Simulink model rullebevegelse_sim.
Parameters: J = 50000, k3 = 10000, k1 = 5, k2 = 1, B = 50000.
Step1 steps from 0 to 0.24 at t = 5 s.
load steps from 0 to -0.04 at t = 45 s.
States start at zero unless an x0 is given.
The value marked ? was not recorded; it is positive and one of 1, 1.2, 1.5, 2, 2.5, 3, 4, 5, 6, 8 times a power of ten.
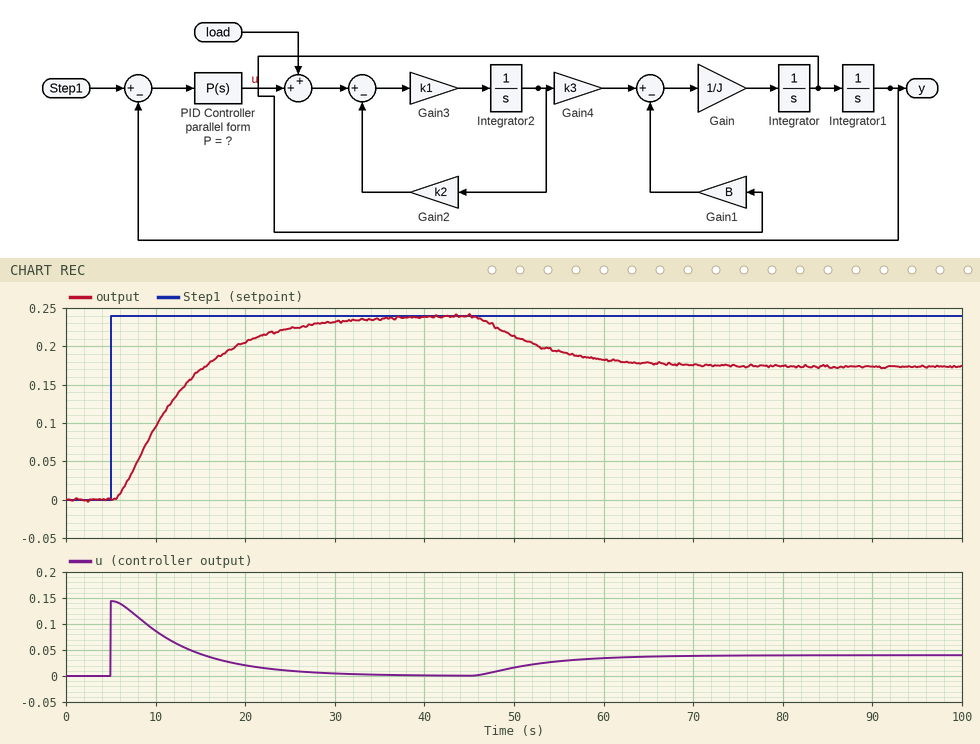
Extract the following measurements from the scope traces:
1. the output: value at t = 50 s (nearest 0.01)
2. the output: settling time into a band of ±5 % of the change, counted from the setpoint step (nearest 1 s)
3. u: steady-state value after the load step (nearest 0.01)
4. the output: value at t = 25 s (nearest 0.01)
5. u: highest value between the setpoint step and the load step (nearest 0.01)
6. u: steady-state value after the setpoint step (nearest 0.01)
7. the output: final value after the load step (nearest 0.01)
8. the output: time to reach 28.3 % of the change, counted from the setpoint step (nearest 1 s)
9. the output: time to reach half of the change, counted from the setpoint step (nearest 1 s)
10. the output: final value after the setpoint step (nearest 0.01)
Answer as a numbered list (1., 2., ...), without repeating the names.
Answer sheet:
1. 0.21
2. 22 s
3. 0.04
4. 0.22
5. 0.14
6. 0.00
7. 0.17
8. 4 s
9. 6 s
10. 0.24
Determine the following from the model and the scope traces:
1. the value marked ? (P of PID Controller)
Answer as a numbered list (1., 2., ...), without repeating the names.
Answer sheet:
1. 0.6
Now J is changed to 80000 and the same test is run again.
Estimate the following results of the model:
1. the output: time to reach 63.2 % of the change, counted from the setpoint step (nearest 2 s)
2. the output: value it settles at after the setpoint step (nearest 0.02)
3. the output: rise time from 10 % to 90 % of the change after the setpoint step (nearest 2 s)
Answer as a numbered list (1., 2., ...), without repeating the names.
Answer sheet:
1. 8 s
2. 0.24
3. 14 s
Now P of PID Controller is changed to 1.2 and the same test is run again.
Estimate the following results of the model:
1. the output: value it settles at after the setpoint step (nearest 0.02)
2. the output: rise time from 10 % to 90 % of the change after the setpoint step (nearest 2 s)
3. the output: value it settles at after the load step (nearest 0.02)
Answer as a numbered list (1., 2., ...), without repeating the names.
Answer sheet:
1. 0.24
2. 6 s
3. 0.20
